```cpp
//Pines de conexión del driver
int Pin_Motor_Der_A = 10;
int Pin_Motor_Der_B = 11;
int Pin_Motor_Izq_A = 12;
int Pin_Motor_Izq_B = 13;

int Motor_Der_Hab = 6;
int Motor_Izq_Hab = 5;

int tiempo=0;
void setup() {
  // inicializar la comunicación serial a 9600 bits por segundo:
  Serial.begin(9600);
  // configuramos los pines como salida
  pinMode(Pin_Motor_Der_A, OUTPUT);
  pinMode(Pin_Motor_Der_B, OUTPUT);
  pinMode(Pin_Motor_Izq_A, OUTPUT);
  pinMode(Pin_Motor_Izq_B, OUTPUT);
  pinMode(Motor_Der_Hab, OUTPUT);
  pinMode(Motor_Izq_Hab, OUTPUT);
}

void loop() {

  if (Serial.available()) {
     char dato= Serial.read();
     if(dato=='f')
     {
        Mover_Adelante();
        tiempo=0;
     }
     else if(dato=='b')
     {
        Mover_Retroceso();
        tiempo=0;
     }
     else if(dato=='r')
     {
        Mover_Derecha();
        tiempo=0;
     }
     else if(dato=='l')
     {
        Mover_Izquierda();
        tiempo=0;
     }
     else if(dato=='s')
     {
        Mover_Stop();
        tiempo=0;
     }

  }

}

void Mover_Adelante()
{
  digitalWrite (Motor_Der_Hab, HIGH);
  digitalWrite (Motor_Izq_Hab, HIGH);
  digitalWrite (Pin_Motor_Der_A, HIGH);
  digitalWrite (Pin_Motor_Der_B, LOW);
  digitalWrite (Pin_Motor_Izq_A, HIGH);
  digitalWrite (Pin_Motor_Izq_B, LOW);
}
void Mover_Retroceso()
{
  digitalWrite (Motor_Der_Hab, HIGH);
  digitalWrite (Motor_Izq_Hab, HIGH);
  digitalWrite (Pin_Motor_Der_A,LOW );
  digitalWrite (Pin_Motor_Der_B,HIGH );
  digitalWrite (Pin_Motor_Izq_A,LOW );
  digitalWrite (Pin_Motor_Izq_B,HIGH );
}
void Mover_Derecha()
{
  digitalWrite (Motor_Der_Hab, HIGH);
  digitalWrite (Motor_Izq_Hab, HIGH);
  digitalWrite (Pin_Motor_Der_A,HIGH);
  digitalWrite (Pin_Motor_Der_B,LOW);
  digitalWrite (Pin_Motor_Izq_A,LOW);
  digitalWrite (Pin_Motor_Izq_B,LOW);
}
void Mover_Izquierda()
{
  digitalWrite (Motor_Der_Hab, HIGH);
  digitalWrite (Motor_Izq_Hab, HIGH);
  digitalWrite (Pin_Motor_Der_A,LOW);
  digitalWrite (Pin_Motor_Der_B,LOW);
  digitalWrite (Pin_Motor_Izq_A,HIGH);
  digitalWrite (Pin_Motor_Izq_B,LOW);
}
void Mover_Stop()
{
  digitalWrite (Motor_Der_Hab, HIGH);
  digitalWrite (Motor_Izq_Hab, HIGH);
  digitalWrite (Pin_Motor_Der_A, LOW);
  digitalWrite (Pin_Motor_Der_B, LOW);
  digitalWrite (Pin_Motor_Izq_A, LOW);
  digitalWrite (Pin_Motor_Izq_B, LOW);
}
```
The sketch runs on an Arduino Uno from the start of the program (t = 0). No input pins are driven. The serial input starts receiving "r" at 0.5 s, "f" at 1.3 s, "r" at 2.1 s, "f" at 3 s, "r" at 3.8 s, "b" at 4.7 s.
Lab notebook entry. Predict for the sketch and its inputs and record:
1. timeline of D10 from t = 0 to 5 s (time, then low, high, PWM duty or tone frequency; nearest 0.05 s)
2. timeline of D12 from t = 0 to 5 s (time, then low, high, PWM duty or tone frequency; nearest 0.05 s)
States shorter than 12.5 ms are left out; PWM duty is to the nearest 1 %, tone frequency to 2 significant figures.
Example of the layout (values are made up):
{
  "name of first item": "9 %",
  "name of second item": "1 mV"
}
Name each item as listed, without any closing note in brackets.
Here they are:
{
  "timeline of D10 from t = 0 to 5 s": "0 s low; 0.5 s high; 4.7 s low",
  "timeline of D12 from t = 0 to 5 s": "0 s low; 1.3 s high; 2.1 s low; 3 s high; 3.8 s low"
}
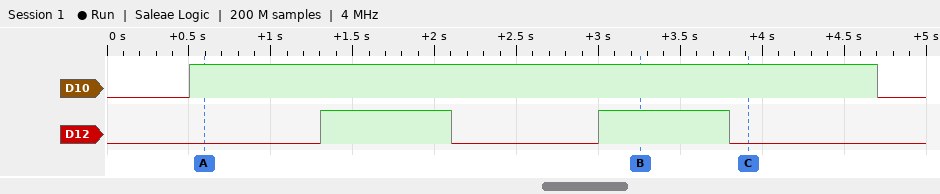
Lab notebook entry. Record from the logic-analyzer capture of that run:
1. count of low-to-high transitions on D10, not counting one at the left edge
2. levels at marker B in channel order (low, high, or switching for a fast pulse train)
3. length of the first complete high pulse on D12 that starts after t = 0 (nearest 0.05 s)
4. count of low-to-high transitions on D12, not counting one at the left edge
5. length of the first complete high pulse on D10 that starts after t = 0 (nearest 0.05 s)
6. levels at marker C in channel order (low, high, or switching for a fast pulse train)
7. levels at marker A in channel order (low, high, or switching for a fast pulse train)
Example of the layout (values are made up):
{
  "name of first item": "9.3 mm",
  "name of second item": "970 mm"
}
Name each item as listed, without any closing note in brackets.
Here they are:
{
  "count of low-to-high transitions on D10, not counting one at the left edge": "1",
  "levels at marker B in channel order": "D10 high, D12 high",
  "length of the first complete high pulse on D12 that starts after t = 0": "0.80 s",
  "count of low-to-high transitions on D12, not counting one at the left edge": "2",
  "length of the first complete high pulse on D10 that starts after t = 0": "4.20 s",
  "levels at marker C in channel order": "D10 high, D12 low",
  "levels at marker A in channel order": "D10 high, D12 low"
}
